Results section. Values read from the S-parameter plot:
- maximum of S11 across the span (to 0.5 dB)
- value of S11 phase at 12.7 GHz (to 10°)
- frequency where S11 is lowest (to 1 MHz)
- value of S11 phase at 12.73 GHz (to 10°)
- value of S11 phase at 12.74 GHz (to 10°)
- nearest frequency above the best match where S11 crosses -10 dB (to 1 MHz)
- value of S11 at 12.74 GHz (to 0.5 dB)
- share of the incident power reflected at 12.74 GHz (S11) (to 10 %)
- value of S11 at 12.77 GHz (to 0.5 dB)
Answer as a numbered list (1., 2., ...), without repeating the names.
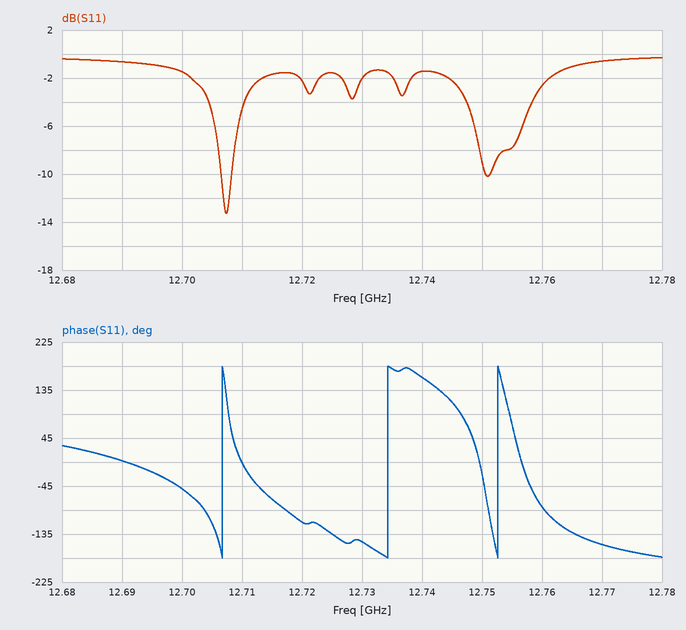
1. -0.5 dB
2. -50°
3. 12.707 GHz
4. -150°
5. 160°
6. 12.708 GHz
7. -1.5 dB
8. 70 %
9. -0.5 dB
